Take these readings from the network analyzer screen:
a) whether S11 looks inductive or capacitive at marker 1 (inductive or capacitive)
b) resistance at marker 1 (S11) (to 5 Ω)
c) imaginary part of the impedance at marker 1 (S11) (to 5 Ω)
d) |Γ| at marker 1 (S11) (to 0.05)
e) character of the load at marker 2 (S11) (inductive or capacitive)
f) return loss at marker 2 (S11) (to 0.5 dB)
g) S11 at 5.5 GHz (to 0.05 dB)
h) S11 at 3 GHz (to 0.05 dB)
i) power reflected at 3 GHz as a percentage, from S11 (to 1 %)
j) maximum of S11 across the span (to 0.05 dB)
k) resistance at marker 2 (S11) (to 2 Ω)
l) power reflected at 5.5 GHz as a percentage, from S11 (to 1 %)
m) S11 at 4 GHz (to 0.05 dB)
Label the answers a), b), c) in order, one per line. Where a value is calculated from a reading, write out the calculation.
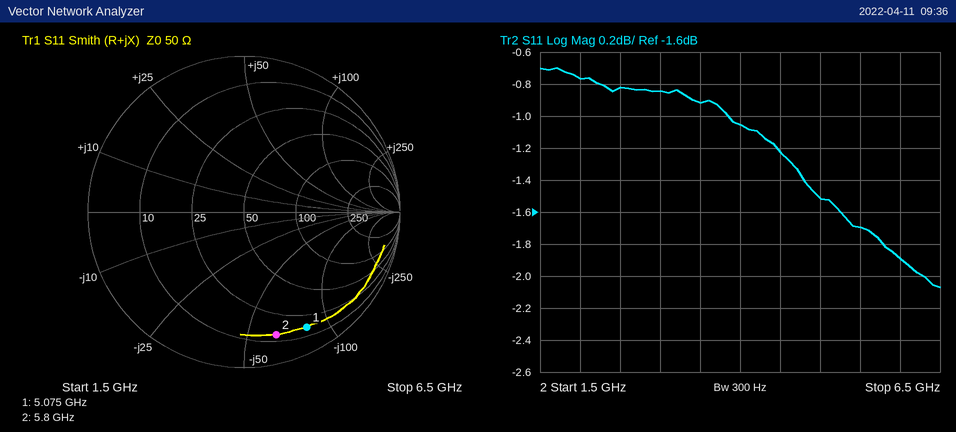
a) capacitive
b) 15 Ω
c) -80 Ω
d) 0.85
e) capacitive
f) 2.0 dB
g) -1.70 dB
h) -0.85 dB
i) 10^(-0.85/10) ≈ 82 %
j) -0.70 dB
k) 14 Ω
l) 10^(-1.7/10) ≈ 68 %
m) -1.05 dB
